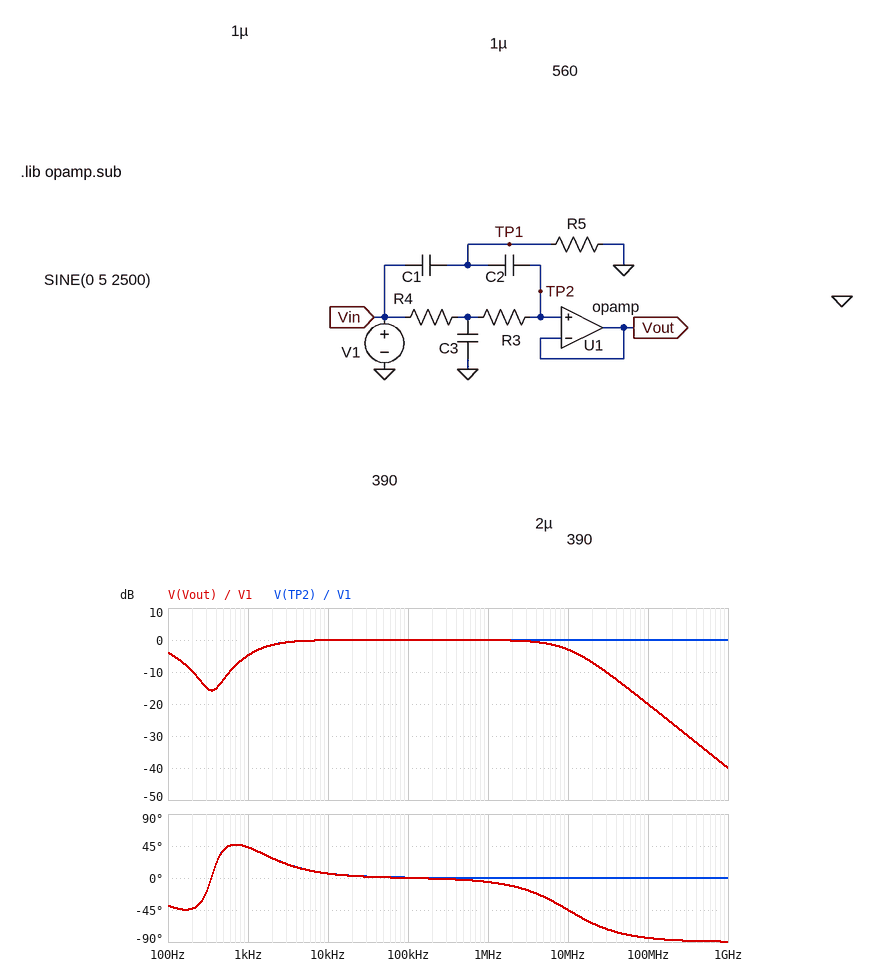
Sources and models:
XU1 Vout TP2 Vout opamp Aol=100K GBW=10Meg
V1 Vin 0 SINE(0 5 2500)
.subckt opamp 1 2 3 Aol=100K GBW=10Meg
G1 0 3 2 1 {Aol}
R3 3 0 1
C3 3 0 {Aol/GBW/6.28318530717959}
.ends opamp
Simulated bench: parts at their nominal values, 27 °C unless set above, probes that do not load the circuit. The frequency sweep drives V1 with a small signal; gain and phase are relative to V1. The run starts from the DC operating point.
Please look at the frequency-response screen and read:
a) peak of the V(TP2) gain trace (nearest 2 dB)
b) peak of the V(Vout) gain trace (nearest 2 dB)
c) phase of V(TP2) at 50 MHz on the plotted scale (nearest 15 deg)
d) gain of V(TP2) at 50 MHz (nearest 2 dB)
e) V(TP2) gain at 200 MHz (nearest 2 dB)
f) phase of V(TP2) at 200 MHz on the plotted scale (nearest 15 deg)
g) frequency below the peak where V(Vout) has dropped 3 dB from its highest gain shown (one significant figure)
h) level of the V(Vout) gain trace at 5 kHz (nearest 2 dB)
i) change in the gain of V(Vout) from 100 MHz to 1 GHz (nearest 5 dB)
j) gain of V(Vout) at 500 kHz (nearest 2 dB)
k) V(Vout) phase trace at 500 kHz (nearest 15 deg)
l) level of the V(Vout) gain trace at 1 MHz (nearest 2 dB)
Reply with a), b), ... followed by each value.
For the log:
a) 0 dB
b) 0 dB
c) 0 deg
d) 0 dB
e) 0 dB
f) 0 deg
g) 1 kHz
h) 0 dB
i) -20 dB
j) 0 dB
k) 0 deg
l) 0 dB
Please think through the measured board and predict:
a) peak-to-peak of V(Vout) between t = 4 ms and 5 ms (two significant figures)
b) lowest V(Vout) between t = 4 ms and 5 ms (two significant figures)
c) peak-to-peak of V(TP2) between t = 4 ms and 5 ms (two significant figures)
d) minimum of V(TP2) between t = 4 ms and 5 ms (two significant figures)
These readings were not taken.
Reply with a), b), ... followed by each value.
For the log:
a) 8.9 V
b) -4.4 V
c) 8.9 V
d) -4.4 V
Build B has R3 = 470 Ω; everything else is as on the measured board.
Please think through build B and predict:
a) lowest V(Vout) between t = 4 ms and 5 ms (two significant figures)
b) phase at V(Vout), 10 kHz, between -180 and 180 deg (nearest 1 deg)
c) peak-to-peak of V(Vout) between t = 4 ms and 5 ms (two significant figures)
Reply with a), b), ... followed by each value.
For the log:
a) -4.5 V
b) 5 deg
c) 9.1 V
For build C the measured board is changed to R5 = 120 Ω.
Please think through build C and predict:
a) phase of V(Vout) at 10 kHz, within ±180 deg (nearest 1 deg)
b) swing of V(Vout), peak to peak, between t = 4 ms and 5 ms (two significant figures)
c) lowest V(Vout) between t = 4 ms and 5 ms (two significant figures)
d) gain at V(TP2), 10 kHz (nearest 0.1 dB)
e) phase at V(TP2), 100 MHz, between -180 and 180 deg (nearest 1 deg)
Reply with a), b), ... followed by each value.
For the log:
a) 12 deg
b) 7.6 V
c) -3.8 V
d) -0.2 dB
e) 0 deg
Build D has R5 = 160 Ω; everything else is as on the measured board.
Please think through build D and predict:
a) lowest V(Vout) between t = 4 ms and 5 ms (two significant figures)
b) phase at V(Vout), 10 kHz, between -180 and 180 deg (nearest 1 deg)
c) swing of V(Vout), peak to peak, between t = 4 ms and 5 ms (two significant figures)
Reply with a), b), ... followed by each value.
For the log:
a) -4.0 V
b) 10 deg
c) 8.1 V
